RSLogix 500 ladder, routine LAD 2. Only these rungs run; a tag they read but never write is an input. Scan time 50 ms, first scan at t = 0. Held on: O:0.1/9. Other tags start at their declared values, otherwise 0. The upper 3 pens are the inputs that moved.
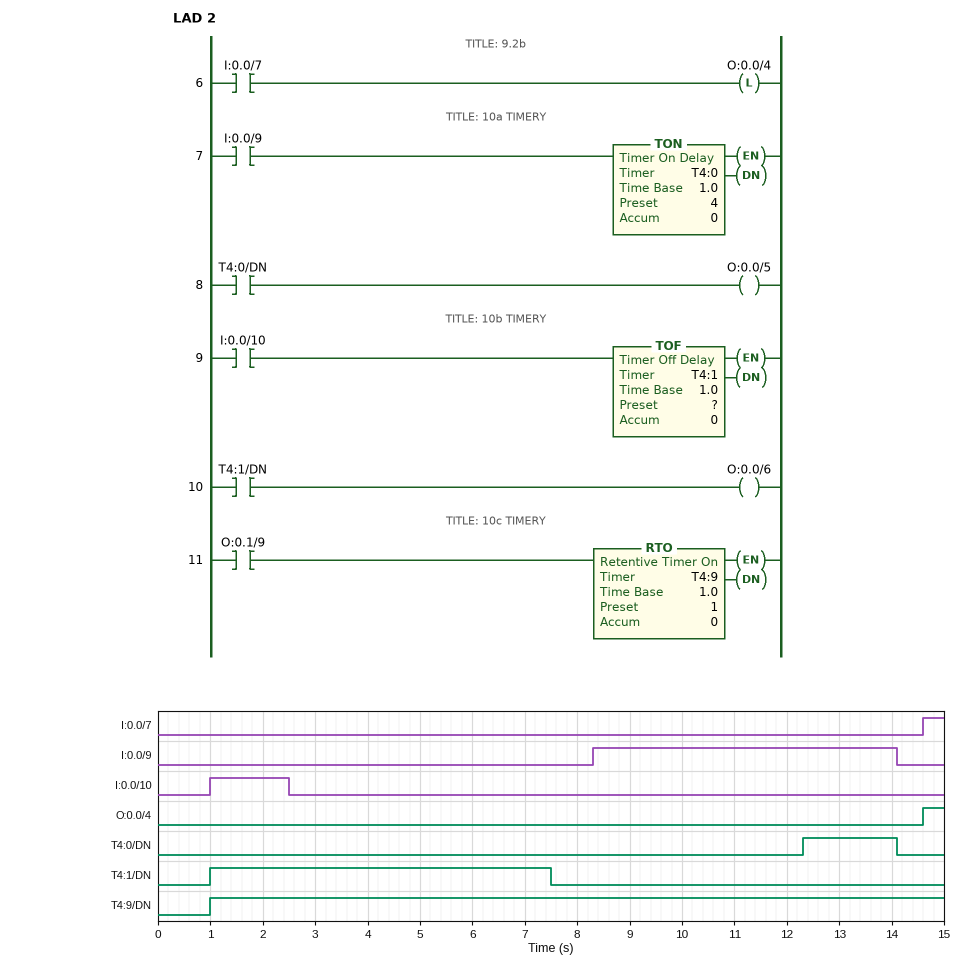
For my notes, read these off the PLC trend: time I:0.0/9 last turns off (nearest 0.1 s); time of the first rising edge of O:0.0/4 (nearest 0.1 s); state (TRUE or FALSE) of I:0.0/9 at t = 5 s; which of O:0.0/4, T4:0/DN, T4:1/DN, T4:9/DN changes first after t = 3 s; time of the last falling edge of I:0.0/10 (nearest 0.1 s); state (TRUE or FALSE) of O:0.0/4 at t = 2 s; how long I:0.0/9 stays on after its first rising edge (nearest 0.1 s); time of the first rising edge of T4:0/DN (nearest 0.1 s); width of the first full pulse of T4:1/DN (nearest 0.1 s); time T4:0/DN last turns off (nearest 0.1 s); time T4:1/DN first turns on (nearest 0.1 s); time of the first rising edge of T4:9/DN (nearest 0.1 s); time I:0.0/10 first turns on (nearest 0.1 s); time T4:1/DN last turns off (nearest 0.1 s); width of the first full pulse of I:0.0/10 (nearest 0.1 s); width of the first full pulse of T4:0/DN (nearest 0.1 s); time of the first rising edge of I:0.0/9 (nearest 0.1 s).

14.1 s
14.6 s
FALSE
T4:1/DN
2.5 s
FALSE
5.8 s
12.3 s
6.5 s
14.1 s
1.0 s
1.0 s
1.0 s
7.5 s
1.5 s
1.8 s
8.3 s
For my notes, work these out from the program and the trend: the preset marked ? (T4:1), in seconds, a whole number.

5 s
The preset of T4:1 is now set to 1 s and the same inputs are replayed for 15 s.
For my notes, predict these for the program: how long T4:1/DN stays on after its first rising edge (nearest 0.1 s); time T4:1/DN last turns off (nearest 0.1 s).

2.5 s
3.5 s
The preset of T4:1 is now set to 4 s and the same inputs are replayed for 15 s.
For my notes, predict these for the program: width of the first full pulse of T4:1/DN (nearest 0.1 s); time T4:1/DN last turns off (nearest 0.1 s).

5.5 s
6.5 s
